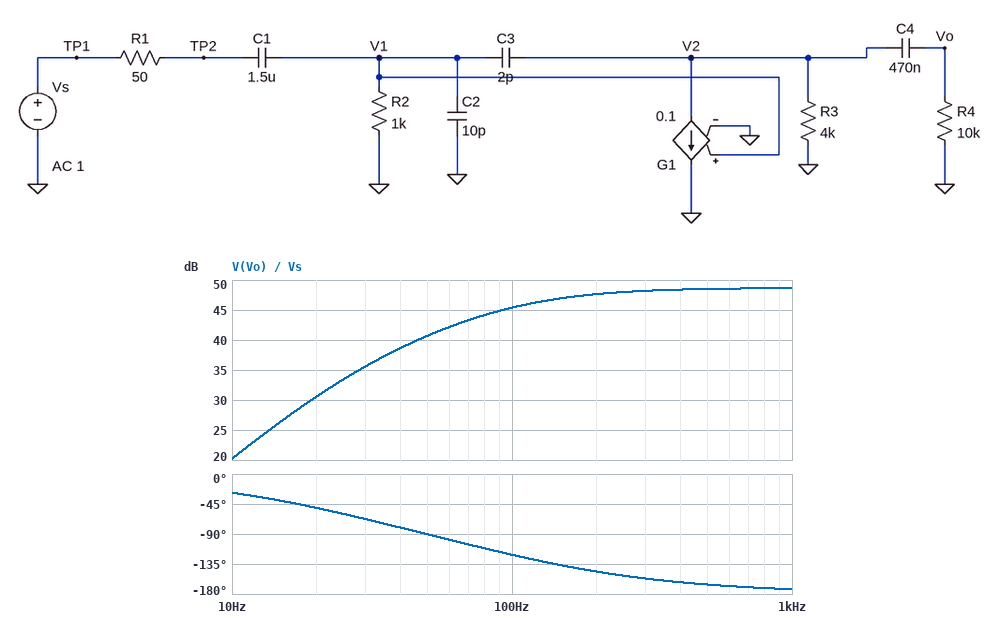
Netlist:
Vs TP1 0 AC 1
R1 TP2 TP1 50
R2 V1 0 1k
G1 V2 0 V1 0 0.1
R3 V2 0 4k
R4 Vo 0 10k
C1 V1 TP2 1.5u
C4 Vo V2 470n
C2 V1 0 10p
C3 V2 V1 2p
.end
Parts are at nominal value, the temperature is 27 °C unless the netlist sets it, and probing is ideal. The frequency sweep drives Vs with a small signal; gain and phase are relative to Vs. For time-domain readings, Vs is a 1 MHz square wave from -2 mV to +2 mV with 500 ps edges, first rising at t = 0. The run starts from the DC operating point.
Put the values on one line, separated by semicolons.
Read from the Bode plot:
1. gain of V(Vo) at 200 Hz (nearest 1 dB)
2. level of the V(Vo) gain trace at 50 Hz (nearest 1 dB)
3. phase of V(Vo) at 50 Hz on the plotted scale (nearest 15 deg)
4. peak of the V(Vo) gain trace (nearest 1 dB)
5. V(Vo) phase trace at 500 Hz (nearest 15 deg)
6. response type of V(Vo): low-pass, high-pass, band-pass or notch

48 dB; 41 dB; -90 deg; 49 dB; -165 deg; high-pass
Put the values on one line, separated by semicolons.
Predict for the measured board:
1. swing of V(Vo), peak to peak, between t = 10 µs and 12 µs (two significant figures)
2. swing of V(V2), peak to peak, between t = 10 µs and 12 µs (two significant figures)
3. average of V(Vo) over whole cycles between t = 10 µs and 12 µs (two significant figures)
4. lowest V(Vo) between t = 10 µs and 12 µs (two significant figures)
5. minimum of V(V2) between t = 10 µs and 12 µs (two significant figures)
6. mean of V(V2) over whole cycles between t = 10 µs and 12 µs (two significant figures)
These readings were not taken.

1.1 V; 1.1 V; -540 mV; -1.1 V; -1.1 V; -540 mV
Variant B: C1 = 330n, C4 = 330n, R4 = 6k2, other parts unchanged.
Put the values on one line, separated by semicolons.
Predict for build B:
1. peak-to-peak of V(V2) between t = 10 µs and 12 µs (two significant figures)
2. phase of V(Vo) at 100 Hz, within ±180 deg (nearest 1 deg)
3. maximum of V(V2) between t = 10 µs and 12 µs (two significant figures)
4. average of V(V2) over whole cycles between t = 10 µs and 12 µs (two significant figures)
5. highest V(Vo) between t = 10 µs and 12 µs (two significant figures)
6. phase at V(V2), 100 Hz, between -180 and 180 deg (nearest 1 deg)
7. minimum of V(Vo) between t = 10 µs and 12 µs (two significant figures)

930 mV; -77 deg; 15 mV; -450 mV; 17 mV; -115 deg; -910 mV
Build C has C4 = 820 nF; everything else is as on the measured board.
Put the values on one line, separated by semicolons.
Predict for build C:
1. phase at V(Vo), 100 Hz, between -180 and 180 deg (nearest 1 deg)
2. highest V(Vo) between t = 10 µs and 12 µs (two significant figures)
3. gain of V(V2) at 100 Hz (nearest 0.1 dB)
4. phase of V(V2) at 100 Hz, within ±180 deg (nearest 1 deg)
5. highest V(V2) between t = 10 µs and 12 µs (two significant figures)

-127 deg; 4.7 mV; 45.7 dB; -138 deg; 3.9 mV
